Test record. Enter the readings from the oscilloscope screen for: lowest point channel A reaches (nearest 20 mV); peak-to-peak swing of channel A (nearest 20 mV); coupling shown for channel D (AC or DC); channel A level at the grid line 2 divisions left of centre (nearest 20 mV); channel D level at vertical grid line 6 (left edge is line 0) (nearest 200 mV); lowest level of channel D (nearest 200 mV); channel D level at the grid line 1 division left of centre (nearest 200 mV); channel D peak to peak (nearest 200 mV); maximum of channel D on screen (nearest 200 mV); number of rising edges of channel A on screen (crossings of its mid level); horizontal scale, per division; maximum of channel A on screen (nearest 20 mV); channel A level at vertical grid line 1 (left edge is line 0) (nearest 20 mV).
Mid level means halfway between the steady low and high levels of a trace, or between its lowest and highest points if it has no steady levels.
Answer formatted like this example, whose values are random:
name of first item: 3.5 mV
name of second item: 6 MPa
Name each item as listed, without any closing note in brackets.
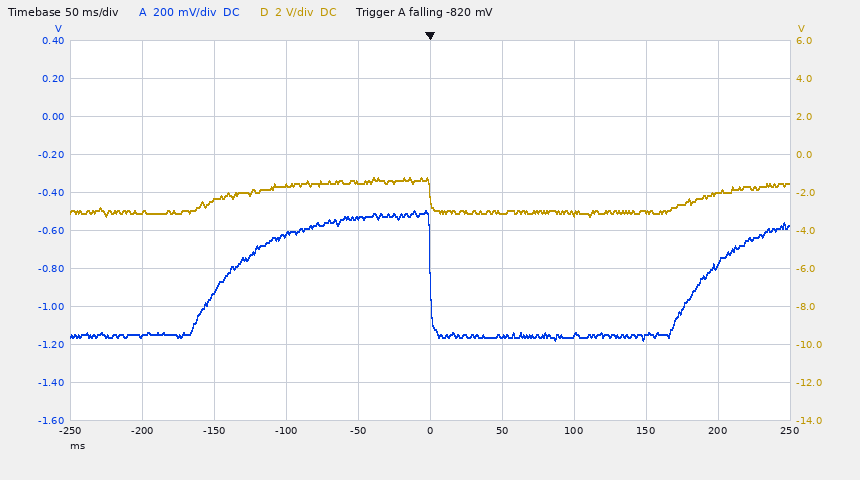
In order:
lowest point channel A reaches: -1.18 V
peak-to-peak swing of channel A: 680 mV
coupling shown for channel D: DC
channel A level at the grid line 2 divisions left of centre: -620 mV
channel D level at vertical grid line 6 (left edge is line 0): -3.0 V
lowest level of channel D: -3.2 V
channel D level at the grid line 1 division left of centre: -1.4 V
channel D peak to peak: 2.0 V
maximum of channel D on screen: -1.2 V
number of rising edges of channel A on screen: 2
horizontal scale, per division: 50 ms
maximum of channel A on screen: -500 mV
channel A level at vertical grid line 1 (left edge is line 0): -1.16 V
